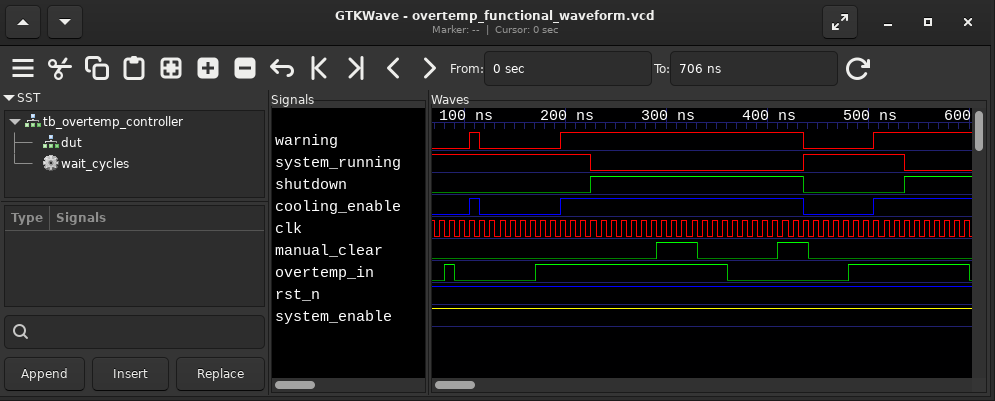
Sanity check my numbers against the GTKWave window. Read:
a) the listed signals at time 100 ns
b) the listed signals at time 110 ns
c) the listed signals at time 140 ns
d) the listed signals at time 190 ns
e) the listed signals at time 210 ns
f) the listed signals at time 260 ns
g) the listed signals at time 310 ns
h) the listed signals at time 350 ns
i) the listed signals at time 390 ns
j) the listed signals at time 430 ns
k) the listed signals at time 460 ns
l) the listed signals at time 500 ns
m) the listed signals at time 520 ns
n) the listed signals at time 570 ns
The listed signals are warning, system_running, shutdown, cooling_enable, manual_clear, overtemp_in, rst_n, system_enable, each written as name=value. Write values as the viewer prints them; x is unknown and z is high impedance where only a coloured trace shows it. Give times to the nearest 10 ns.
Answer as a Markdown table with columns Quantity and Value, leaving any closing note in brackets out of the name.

| Quantity | Value |
|---|---|
| the listed signals at time 100 ns | warning=0, system_running=1, shutdown=0, cooling_enable=0, manual_clear=0, overtemp_in=0, rst_n=1, system_enable=1 |
| the listed signals at time 110 ns | warning=1, system_running=1, shutdown=0, cooling_enable=1, manual_clear=0, overtemp_in=0, rst_n=1, system_enable=1 |
| the listed signals at time 140 ns | warning=0, system_running=1, shutdown=0, cooling_enable=0, manual_clear=0, overtemp_in=0, rst_n=1, system_enable=1 |
| the listed signals at time 190 ns | warning=0, system_running=1, shutdown=0, cooling_enable=0, manual_clear=0, overtemp_in=1, rst_n=1, system_enable=1 |
| the listed signals at time 210 ns | warning=1, system_running=1, shutdown=0, cooling_enable=1, manual_clear=0, overtemp_in=1, rst_n=1, system_enable=1 |
| the listed signals at time 260 ns | warning=1, system_running=0, shutdown=1, cooling_enable=1, manual_clear=0, overtemp_in=1, rst_n=1, system_enable=1 |
| the listed signals at time 310 ns | warning=1, system_running=0, shutdown=1, cooling_enable=1, manual_clear=1, overtemp_in=1, rst_n=1, system_enable=1 |
| the listed signals at time 350 ns | warning=1, system_running=0, shutdown=1, cooling_enable=1, manual_clear=0, overtemp_in=1, rst_n=1, system_enable=1 |
| the listed signals at time 390 ns | warning=1, system_running=0, shutdown=1, cooling_enable=1, manual_clear=0, overtemp_in=0, rst_n=1, system_enable=1 |
| the listed signals at time 430 ns | warning=1, system_running=0, shutdown=1, cooling_enable=1, manual_clear=1, overtemp_in=0, rst_n=1, system_enable=1 |
| the listed signals at time 460 ns | warning=0, system_running=1, shutdown=0, cooling_enable=0, manual_clear=0, overtemp_in=0, rst_n=1, system_enable=1 |
| the listed signals at time 500 ns | warning=0, system_running=1, shutdown=0, cooling_enable=0, manual_clear=0, overtemp_in=1, rst_n=1, system_enable=1 |
| the listed signals at time 520 ns | warning=1, system_running=1, shutdown=0, cooling_enable=1, manual_clear=0, overtemp_in=1, rst_n=1, system_enable=1 |
| the listed signals at time 570 ns | warning=1, system_running=0, shutdown=1, cooling_enable=1, manual_clear=0, overtemp_in=1, rst_n=1, system_enable=1 |
